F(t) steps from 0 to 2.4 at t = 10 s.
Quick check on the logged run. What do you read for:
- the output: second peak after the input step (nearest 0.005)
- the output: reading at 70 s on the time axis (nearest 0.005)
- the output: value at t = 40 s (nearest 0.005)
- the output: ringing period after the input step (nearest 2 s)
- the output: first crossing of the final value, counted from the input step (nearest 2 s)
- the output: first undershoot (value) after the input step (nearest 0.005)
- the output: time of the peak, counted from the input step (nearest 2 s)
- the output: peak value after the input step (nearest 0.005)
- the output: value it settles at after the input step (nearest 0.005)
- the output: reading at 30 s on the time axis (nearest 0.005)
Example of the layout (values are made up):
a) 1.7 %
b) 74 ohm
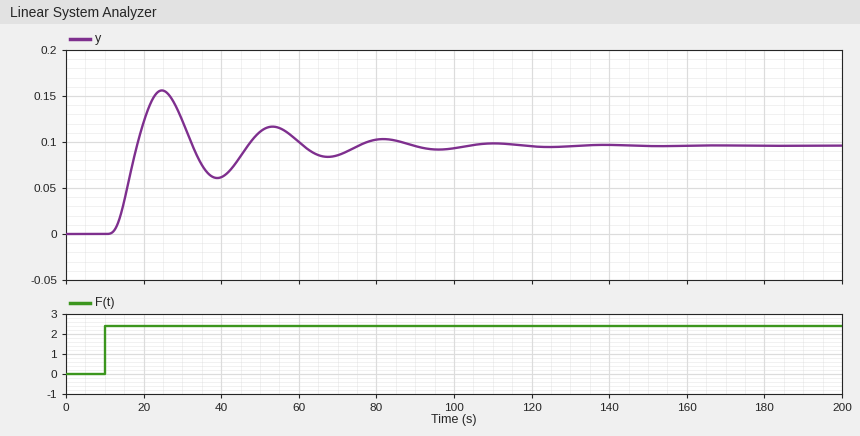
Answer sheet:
a) 0.115
b) 0.085
c) 0.060
d) 28 s
e) 8 s
f) 0.060
g) 14 s
h) 0.155
i) 0.095
j) 0.125
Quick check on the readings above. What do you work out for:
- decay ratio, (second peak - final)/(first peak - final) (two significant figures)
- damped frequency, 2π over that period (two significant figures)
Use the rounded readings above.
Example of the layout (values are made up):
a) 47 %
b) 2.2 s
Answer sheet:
a) 0.33
b) 0.22 rad/s
